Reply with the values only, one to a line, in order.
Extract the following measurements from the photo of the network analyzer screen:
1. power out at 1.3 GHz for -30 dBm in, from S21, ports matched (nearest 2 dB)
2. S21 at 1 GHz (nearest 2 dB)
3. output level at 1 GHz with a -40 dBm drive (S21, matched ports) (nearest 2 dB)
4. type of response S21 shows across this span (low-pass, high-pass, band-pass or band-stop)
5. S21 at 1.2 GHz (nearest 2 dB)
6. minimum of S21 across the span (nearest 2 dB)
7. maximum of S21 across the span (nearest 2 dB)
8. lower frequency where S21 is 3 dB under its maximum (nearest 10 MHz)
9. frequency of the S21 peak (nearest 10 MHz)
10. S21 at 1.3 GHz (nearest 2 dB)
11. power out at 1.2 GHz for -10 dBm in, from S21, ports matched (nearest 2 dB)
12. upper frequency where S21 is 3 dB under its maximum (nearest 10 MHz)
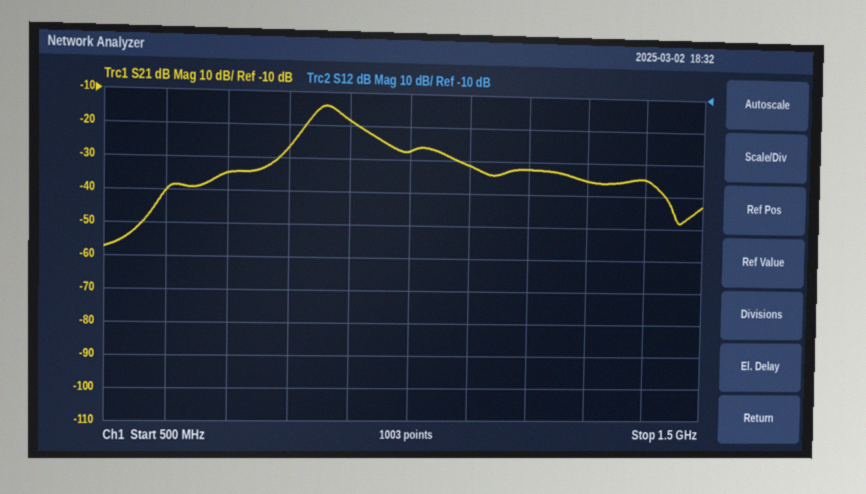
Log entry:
-66 dBm
-28 dB
-68 dBm
band-pass
-32 dB
-58 dB
-14 dB
840 MHz
860 MHz
-36 dB
-42 dBm
890 MHz
